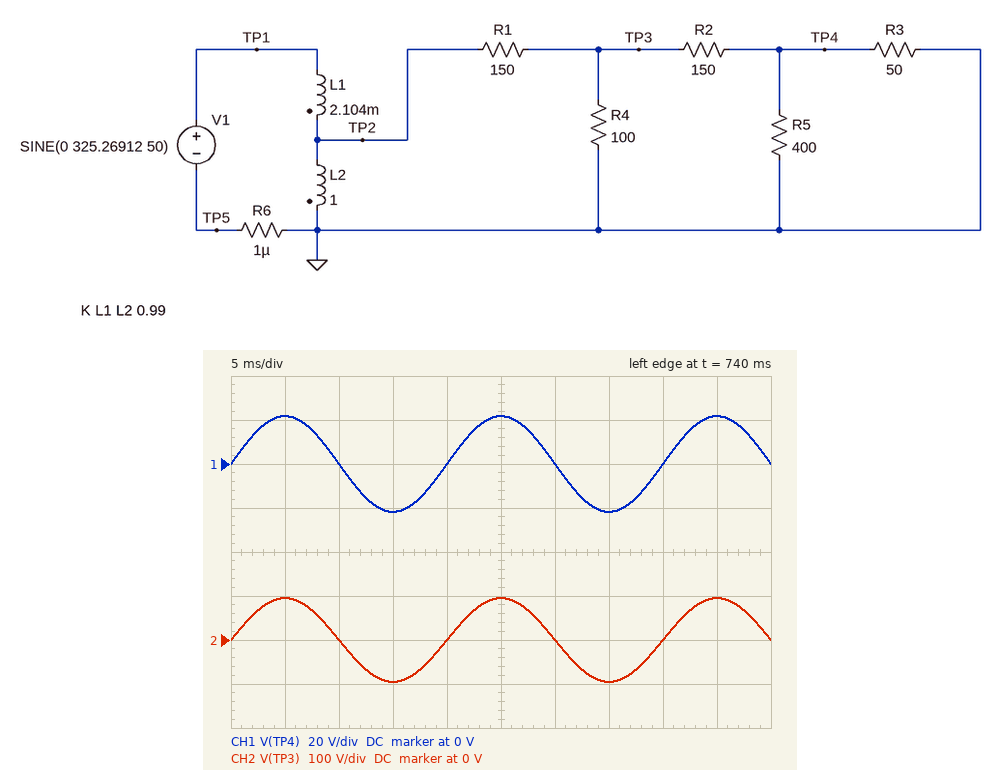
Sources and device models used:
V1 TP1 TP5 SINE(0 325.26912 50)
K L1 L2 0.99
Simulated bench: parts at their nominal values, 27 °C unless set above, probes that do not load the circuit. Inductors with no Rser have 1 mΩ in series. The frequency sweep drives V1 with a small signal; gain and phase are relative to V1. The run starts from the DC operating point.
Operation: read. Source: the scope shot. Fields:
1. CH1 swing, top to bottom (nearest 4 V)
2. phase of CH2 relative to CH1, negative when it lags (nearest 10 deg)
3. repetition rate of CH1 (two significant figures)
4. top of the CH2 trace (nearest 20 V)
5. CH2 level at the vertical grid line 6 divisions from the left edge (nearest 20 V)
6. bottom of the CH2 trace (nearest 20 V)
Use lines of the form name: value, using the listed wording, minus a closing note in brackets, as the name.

CH1 swing, top to bottom: 44 V
phase of CH2 relative to CH1, negative when it lags: 0 deg
repetition rate of CH1: 50 Hz
top of the CH2 trace: 100 V
CH2 level at the vertical grid line 6 divisions from the left edge: 0 V
bottom of the CH2 trace: -100 V
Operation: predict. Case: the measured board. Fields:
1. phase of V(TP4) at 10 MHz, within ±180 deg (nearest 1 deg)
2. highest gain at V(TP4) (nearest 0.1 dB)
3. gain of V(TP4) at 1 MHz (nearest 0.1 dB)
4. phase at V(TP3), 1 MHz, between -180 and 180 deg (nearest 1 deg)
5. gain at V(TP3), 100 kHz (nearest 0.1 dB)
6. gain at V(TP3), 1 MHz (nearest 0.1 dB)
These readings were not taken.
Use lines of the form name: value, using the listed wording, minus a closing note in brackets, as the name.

phase of V(TP4) at 10 MHz, within ±180 deg: -85 deg
highest gain at V(TP4): -23.5 dB
gain of V(TP4) at 1 MHz: -27.0 dB
phase at V(TP3), 1 MHz, between -180 and 180 deg: -48 deg
gain at V(TP3), 100 kHz: -10.7 dB
gain at V(TP3), 1 MHz: -14.2 dB
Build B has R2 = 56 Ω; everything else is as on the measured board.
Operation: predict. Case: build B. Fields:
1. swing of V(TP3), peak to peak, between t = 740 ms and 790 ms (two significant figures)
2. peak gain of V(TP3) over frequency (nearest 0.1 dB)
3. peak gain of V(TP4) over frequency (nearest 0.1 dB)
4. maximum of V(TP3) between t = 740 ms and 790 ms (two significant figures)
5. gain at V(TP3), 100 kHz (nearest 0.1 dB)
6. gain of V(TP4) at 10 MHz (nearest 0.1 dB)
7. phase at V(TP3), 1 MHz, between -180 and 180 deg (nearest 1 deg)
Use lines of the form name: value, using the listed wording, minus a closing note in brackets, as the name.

swing of V(TP3), peak to peak, between t = 740 ms and 790 ms: 160 V
peak gain of V(TP3) over frequency: -12.4 dB
peak gain of V(TP4) over frequency: -19.5 dB
maximum of V(TP3) between t = 740 ms and 790 ms: 78 V
gain at V(TP3), 100 kHz: -12.5 dB
gain of V(TP4) at 10 MHz: -41.1 dB
phase at V(TP3), 1 MHz, between -180 and 180 deg: -50 deg
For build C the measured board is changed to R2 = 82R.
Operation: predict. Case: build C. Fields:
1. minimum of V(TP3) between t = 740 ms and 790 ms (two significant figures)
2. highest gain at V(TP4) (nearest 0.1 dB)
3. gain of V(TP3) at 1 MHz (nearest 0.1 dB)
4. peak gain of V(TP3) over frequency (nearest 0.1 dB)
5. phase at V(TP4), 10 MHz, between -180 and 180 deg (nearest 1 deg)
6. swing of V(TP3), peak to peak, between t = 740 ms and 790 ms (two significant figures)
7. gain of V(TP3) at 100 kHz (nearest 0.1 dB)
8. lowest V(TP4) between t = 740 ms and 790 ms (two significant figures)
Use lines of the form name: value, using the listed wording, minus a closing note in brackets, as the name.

minimum of V(TP3) between t = 740 ms and 790 ms: -84 V
highest gain at V(TP4): -20.8 dB
gain of V(TP3) at 1 MHz: -15.5 dB
peak gain of V(TP3) over frequency: -11.7 dB
phase at V(TP4), 10 MHz, between -180 and 180 deg: -85 deg
swing of V(TP3), peak to peak, between t = 740 ms and 790 ms: 170 V
gain of V(TP3) at 100 kHz: -11.8 dB
lowest V(TP4) between t = 740 ms and 790 ms: -30 V
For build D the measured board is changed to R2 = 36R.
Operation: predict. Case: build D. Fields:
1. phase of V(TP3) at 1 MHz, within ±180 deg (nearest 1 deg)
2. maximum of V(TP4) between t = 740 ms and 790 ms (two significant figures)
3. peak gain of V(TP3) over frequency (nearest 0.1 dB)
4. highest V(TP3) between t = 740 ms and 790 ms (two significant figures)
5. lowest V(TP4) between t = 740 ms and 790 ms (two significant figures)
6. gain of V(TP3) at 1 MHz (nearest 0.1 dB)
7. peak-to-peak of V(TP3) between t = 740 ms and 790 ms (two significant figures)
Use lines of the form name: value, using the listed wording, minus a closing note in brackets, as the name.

phase of V(TP3) at 1 MHz, within ±180 deg: -51 deg
maximum of V(TP4) between t = 740 ms and 790 ms: 39 V
peak gain of V(TP3) over frequency: -13.2 dB
highest V(TP3) between t = 740 ms and 790 ms: 71 V
lowest V(TP4) between t = 740 ms and 790 ms: -39 V
gain of V(TP3) at 1 MHz: -17.2 dB
peak-to-peak of V(TP3) between t = 740 ms and 790 ms: 140 V
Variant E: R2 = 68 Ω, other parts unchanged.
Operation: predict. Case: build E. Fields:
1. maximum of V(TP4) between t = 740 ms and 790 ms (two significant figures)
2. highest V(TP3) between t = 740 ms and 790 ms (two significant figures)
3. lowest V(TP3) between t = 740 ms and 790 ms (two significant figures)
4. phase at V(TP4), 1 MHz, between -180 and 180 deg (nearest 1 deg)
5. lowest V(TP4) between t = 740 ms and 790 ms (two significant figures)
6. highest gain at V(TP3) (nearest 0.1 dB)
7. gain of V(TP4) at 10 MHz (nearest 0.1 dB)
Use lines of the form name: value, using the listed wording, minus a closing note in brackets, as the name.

maximum of V(TP4) between t = 740 ms and 790 ms: 32 V
highest V(TP3) between t = 740 ms and 790 ms: 81 V
lowest V(TP3) between t = 740 ms and 790 ms: -81 V
phase at V(TP4), 1 MHz, between -180 and 180 deg: -50 deg
lowest V(TP4) between t = 740 ms and 790 ms: -32 V
highest gain at V(TP3): -12.1 dB
gain of V(TP4) at 10 MHz: -41.6 dB
